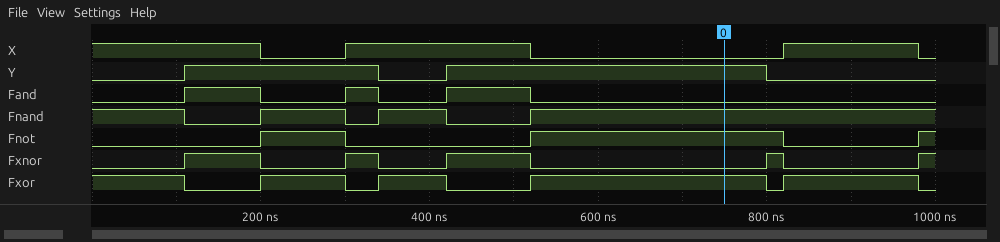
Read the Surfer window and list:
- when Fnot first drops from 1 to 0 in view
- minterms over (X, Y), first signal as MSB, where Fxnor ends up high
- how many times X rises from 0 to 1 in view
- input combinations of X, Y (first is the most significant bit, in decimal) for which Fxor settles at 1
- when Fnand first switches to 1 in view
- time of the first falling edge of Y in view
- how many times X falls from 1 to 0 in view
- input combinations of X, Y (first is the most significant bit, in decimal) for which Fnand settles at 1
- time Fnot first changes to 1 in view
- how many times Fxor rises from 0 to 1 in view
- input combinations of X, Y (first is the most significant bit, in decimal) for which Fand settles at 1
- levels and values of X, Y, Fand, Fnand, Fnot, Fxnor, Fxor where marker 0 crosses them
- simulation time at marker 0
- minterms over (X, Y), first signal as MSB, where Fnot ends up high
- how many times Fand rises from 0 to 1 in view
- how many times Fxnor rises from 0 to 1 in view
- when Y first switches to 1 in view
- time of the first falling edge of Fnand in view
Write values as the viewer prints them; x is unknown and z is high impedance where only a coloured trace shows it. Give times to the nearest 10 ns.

300 ns
0, 3
2
1, 2
200 ns
340 ns
3
0, 1, 2
200 ns
4
3
X=0, Y=1, Fand=0, Fnand=1, Fnot=1, Fxnor=0, Fxor=1
750 ns
0, 1
3
5
110 ns
110 ns
